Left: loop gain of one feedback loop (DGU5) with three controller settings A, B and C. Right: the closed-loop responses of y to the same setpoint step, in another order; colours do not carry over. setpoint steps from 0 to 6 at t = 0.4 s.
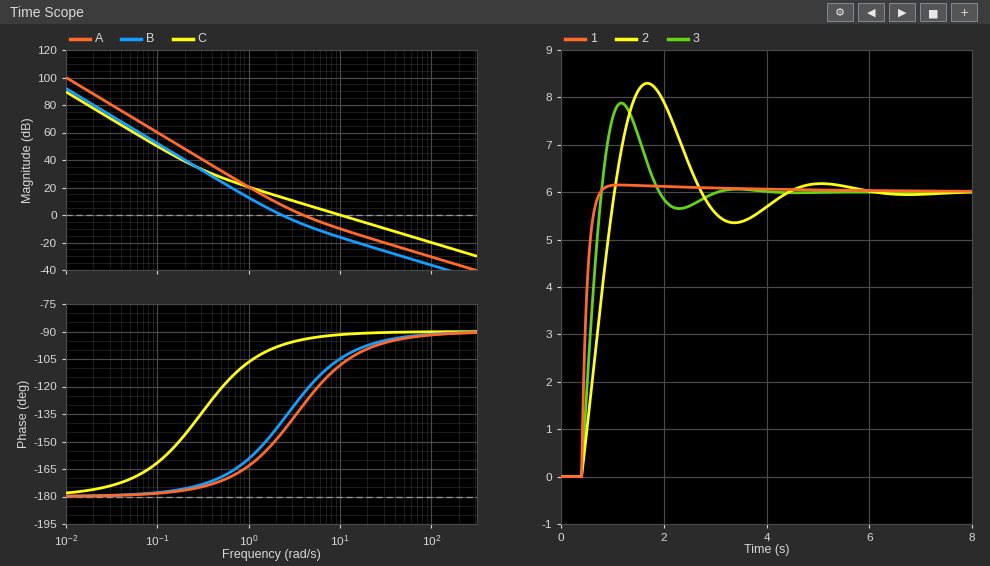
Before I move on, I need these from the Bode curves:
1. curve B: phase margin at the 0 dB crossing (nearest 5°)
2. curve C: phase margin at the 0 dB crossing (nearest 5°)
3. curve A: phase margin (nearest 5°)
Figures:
40°
90°
50°
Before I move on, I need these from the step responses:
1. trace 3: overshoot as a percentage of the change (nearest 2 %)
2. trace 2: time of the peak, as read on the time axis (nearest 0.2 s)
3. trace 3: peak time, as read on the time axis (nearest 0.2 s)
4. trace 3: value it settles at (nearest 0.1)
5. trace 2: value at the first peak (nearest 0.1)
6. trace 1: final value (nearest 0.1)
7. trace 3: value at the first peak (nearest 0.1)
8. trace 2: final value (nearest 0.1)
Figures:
32 %
1.6 s
1.2 s
6.0
8.3
6.0
7.9
6.0
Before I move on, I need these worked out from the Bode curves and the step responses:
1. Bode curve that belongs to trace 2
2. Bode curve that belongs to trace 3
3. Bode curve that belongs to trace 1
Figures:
B
A
C
